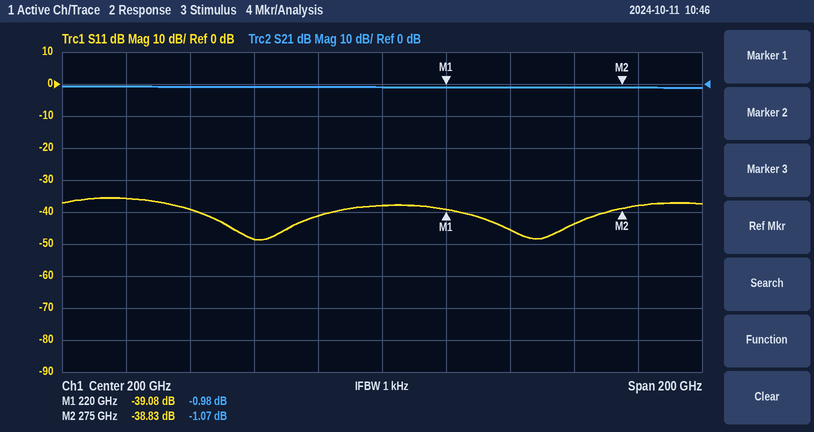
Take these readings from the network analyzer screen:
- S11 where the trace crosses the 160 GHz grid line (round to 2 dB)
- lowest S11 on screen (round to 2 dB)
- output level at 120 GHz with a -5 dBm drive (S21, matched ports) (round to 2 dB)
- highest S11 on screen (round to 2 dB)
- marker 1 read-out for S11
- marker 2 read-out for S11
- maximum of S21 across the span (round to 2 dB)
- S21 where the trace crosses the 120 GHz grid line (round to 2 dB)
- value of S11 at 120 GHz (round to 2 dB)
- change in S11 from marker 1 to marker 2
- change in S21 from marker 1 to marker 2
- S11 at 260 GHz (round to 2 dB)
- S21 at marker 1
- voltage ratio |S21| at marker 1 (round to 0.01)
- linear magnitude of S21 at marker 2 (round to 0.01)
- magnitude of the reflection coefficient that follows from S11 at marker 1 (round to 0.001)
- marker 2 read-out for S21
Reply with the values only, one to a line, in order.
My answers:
-48 dB
-48 dB
-6 dBm
-36 dB
-39.08 dB
-38.83 dB
0 dB
0 dB
-36 dB
0.25 dB
-0.09 dB
-44 dB
-0.98 dB
0.89
0.88
0.011
-1.07 dB
